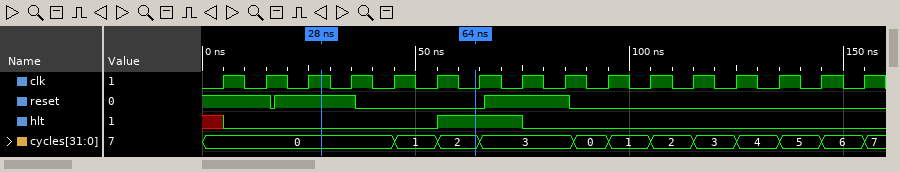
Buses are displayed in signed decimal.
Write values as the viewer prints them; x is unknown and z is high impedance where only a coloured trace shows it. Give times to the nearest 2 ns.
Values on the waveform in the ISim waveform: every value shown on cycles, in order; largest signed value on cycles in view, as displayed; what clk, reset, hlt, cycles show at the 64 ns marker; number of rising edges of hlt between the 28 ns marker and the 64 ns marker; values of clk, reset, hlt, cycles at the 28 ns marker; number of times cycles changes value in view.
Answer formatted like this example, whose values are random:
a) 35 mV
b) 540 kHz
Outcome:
a) 0, 1, 2, 3, 0, 1, 2, 3, 4, 5, 6, 7
b) 7
c) clk=0, reset=0, hlt=1, cycles=2
d) 1
e) clk=1, reset=1, hlt=0, cycles=0
f) 11
